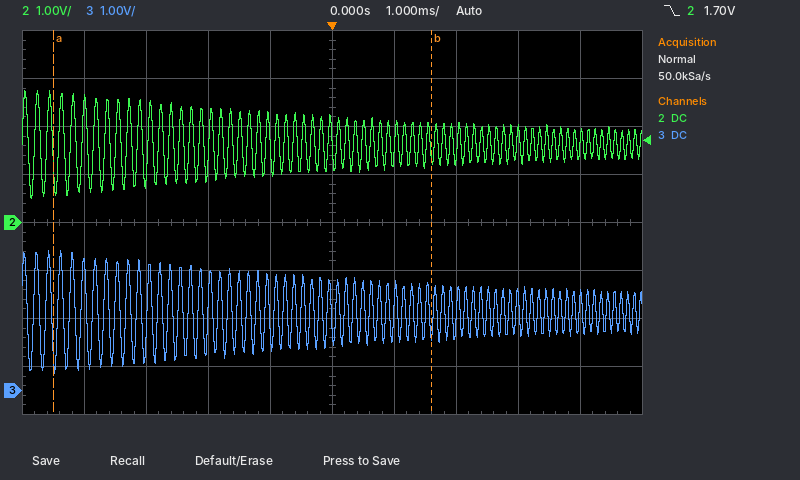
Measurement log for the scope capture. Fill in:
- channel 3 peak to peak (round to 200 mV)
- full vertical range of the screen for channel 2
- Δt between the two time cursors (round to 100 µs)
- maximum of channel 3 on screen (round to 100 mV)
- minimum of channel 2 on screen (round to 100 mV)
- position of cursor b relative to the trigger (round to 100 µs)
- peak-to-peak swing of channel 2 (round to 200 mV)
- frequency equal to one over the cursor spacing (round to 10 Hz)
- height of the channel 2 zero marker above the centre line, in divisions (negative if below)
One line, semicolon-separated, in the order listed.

2.6 V; 8 V; 6.1 ms; 2.9 V; 500 mV; +1.6 ms; 2.2 V; 160 Hz; 0.0 div
